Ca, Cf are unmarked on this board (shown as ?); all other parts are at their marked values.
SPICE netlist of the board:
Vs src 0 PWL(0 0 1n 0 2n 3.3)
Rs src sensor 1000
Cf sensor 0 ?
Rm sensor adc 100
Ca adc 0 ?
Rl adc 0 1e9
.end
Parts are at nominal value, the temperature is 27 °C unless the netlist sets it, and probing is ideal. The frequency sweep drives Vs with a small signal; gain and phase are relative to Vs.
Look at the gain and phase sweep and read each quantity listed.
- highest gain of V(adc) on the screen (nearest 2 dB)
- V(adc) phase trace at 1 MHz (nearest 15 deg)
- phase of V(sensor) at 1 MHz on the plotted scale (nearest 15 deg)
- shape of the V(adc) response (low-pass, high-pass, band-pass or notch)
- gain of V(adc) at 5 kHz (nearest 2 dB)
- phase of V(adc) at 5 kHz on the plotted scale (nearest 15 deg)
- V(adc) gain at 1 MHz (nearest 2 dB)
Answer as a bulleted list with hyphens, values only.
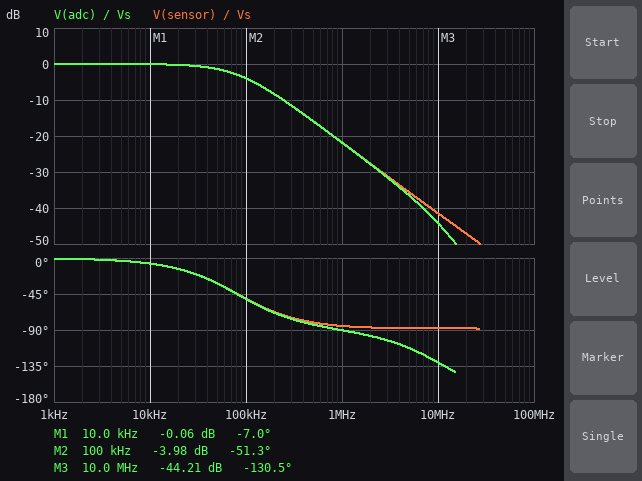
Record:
- 0 dB
- -90 deg
- -90 deg
- low-pass
- 0 dB
- 0 deg
- -22 dB
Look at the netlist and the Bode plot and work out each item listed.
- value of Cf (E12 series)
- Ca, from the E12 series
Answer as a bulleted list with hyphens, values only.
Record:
- 1.8 nF
- 150 pF
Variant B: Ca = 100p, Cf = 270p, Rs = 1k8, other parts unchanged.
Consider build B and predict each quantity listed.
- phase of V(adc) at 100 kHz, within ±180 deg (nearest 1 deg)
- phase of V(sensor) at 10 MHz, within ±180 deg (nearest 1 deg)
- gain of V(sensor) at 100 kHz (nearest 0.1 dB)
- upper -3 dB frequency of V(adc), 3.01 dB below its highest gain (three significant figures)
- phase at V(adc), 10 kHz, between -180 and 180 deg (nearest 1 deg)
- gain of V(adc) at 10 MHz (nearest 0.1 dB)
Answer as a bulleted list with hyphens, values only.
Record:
- -23 deg
- -81 deg
- -0.7 dB
- 238 kHz
- -2 deg
- -33.3 dB
